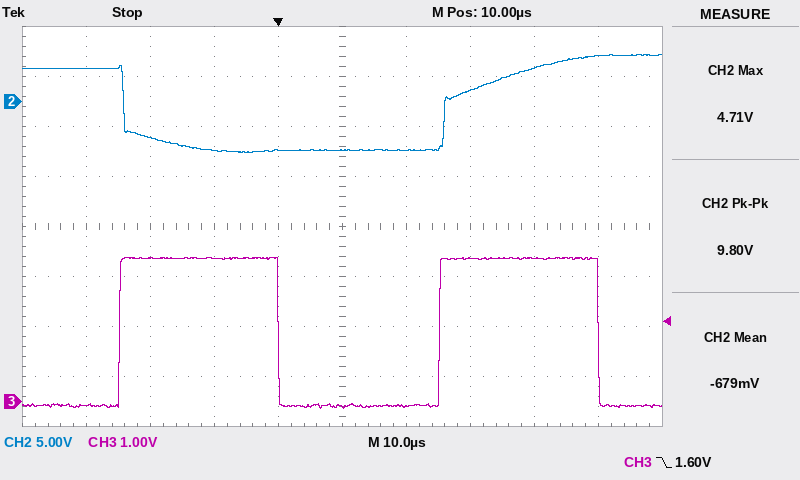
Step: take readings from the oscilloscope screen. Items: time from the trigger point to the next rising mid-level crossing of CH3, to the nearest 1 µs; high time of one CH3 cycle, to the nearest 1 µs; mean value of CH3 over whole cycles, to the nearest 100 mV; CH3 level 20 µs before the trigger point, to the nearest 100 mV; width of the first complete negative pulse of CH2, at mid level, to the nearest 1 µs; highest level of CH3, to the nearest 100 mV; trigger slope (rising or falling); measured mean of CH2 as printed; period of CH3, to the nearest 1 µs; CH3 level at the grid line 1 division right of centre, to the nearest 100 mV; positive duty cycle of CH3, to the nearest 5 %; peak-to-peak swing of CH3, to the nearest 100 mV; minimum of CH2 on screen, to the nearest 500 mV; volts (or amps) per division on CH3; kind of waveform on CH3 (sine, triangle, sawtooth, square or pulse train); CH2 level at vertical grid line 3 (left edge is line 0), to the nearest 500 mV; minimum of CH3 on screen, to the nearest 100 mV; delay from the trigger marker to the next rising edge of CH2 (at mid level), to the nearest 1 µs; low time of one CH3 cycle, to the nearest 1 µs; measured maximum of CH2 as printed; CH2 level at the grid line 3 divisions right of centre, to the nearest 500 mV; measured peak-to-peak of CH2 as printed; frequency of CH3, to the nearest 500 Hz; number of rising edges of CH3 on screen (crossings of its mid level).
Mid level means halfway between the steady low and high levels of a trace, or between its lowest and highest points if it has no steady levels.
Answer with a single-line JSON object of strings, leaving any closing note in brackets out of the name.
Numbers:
{"time from the trigger point to the next rising mid-level crossing of CH3, to the nearest 1 µs": "25 µs", "high time of one CH3 cycle, to the nearest 1 µs": "25 µs", "mean value of CH3 over whole cycles, to the nearest 100 mV": "1.4 V", "CH3 level 20 µs before the trigger point, to the nearest 100 mV": "2.9 V", "width of the first complete negative pulse of CH2, at mid level, to the nearest 1 µs": "50 µs", "highest level of CH3, to the nearest 100 mV": "2.9 V", "trigger slope": "falling", "measured mean of CH2 as printed": "-679 mV", "period of CH3, to the nearest 1 µs": "50 µs", "CH3 level at the grid line 1 division right of centre, to the nearest 100 mV": "-100 mV", "positive duty cycle of CH3, to the nearest 5 %": "50 %", "peak-to-peak swing of CH3, to the nearest 100 mV": "3.0 V", "minimum of CH2 on screen, to the nearest 500 mV": "-5.0 V", "volts (or amps) per division on CH3": "1 V", "kind of waveform on CH3": "square", "CH2 level at vertical grid line 3 (left edge is line 0), to the nearest 500 mV": "-5.0 V", "minimum of CH3 on screen, to the nearest 100 mV": "-100 mV", "delay from the trigger marker to the next rising edge of CH2 (at mid level), to the nearest 1 µs": "26 µs", "low time of one CH3 cycle, to the nearest 1 µs": "25 µs", "measured maximum of CH2 as printed": "4.71 V", "CH2 level at the grid line 3 divisions right of centre, to the nearest 500 mV": "3.5 V", "measured peak-to-peak of CH2 as printed": "9.80 V", "frequency of CH3, to the nearest 500 Hz": "20.0 kHz", "number of rising edges of CH3 on screen": "2"}
